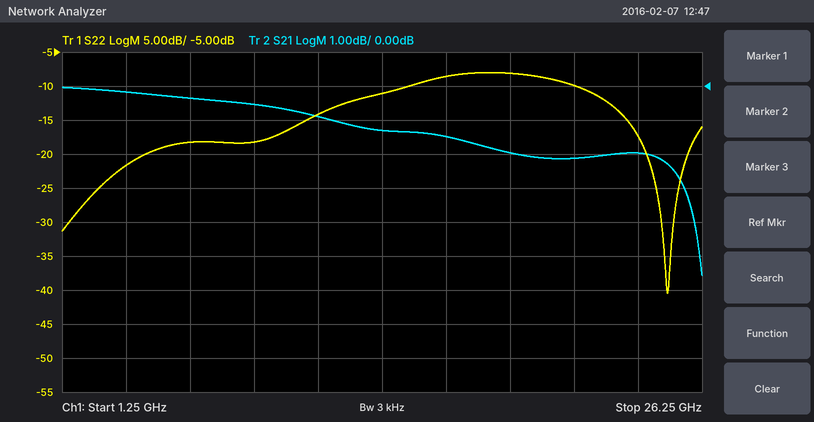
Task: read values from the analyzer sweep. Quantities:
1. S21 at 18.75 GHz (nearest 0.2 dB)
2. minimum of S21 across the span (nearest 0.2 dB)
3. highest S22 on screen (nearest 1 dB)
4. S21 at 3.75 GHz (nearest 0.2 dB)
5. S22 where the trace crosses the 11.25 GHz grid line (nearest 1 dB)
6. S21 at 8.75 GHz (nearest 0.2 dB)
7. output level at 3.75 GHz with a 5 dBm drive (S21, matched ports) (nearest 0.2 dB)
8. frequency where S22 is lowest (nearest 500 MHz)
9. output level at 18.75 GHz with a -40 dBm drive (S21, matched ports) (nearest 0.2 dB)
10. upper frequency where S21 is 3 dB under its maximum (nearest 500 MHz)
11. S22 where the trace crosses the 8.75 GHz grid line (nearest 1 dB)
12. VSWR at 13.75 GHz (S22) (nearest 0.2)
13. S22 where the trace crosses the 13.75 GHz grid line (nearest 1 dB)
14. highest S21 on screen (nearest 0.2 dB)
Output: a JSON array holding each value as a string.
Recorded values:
["-2.0 dB", "-5.6 dB", "-8 dB", "-0.2 dB", "-14 dB", "-0.6 dB", "4.8 dBm", "25.0 GHz", "-42.0 dBm", "25.5 GHz", "-18 dB", "1.8", "-11 dB", "0.0 dB"]
